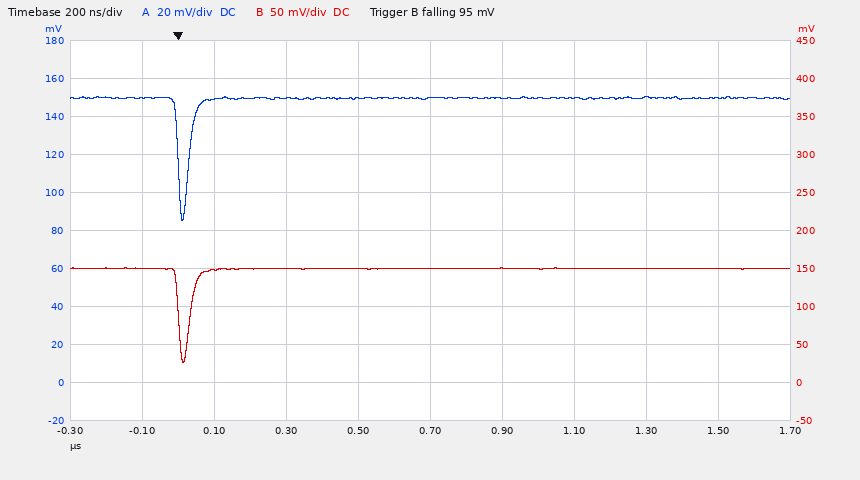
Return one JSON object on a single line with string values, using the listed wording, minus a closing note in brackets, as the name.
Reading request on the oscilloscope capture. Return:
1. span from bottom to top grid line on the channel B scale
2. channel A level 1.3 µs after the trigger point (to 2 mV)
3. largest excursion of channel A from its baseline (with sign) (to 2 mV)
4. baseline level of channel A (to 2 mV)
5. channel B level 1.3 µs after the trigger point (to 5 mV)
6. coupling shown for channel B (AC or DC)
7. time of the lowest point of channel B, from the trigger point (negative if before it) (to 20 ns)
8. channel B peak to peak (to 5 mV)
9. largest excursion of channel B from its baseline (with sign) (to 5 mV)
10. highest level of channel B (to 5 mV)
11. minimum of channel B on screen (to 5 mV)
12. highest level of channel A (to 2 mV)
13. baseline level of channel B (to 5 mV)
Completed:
{"span from bottom to top grid line on the channel B scale": "500 mV", "channel A level 1.3 µs after the trigger point": "150 mV", "largest excursion of channel A from its baseline (with sign)": "-64 mV", "baseline level of channel A": "150 mV", "channel B level 1.3 µs after the trigger point": "150 mV", "coupling shown for channel B": "DC", "time of the lowest point of channel B, from the trigger point (negative if before it)": "+20 ns", "channel B peak to peak": "125 mV", "largest excursion of channel B from its baseline (with sign)": "-125 mV", "highest level of channel B": "150 mV", "minimum of channel B on screen": "25 mV", "highest level of channel A": "150 mV", "baseline level of channel B": "150 mV"}
